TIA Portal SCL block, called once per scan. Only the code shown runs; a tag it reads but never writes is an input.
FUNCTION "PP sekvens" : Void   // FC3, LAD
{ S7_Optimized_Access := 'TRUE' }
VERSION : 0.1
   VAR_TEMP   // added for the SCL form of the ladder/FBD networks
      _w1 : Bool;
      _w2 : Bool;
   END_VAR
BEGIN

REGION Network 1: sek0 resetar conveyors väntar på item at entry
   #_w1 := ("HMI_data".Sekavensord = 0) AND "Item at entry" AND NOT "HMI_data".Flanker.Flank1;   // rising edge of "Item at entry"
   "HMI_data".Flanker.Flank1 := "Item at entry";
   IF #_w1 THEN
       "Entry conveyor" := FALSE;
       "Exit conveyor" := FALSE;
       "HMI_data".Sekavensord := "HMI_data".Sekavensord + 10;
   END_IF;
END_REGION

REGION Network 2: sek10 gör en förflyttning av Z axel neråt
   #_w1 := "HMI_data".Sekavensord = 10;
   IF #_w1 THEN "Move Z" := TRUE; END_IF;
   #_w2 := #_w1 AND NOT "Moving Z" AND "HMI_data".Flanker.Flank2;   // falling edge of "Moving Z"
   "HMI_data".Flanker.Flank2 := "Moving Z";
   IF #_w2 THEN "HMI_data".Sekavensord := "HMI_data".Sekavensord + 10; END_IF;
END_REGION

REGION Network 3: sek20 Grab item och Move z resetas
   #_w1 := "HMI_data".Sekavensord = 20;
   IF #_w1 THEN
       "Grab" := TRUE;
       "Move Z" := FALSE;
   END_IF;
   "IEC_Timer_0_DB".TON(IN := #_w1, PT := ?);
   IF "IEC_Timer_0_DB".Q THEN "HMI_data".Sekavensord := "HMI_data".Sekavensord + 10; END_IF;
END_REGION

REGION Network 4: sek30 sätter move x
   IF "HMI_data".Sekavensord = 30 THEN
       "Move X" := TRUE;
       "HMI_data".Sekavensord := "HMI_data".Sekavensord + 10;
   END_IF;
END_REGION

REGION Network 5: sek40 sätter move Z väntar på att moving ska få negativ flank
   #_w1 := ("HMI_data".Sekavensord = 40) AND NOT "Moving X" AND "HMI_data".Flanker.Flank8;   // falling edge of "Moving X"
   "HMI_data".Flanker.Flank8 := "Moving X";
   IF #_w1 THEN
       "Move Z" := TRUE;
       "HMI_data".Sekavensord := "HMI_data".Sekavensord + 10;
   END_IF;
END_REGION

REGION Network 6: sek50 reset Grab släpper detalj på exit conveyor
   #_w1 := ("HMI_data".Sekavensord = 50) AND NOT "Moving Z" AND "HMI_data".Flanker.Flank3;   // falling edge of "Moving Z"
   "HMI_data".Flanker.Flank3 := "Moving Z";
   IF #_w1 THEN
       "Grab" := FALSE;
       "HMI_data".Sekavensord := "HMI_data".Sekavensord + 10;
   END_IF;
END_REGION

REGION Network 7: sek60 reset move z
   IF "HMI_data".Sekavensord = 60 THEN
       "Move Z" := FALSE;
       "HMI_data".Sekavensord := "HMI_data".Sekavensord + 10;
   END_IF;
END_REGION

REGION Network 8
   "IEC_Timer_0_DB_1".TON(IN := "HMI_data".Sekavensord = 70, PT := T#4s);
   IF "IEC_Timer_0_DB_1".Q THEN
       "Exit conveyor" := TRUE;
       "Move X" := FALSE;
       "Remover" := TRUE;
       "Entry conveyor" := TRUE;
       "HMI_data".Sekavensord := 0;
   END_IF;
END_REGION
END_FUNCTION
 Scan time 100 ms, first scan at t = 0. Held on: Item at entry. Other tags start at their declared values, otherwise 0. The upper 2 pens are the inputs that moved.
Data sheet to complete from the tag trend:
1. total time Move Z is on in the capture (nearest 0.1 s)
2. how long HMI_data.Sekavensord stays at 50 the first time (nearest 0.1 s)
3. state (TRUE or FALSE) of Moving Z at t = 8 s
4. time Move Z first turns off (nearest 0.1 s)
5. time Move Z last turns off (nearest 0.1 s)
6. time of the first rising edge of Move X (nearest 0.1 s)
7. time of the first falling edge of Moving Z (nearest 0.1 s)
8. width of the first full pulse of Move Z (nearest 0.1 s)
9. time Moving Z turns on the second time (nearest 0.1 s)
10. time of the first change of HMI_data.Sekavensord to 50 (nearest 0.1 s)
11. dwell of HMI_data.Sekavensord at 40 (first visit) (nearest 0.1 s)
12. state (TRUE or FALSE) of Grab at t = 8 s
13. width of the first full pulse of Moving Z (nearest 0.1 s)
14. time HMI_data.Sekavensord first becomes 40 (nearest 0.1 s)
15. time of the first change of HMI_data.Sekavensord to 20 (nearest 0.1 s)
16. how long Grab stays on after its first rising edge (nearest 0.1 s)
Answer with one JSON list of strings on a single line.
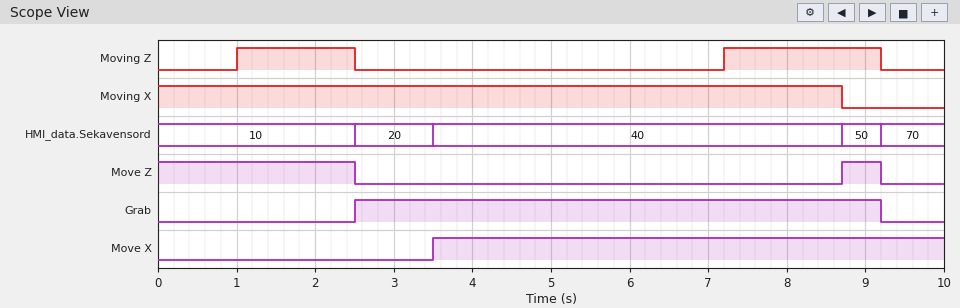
["3.0 s", "0.5 s", "TRUE", "2.5 s", "9.2 s", "3.5 s", "2.5 s", "0.5 s", "7.2 s", "8.7 s", "5.2 s", "TRUE", "1.5 s", "3.5 s", "2.5 s", "6.7 s"]
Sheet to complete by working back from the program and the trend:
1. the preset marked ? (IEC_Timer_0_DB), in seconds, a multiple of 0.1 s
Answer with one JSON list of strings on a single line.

["1.0 s"]
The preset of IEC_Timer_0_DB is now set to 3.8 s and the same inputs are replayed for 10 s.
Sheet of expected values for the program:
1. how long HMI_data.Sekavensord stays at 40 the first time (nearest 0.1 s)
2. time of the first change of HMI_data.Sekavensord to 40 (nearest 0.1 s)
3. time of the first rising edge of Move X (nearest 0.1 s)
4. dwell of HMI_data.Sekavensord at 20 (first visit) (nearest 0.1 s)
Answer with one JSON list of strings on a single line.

["2.4 s", "6.3 s", "6.3 s", "3.8 s"]
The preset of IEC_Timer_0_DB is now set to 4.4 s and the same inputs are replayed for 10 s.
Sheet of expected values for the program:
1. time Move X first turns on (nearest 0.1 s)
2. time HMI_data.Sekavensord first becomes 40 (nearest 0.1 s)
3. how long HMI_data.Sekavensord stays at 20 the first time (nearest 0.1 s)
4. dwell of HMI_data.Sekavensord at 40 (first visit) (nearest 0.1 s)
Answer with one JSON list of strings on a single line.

["6.9 s", "6.9 s", "4.4 s", "1.8 s"]
